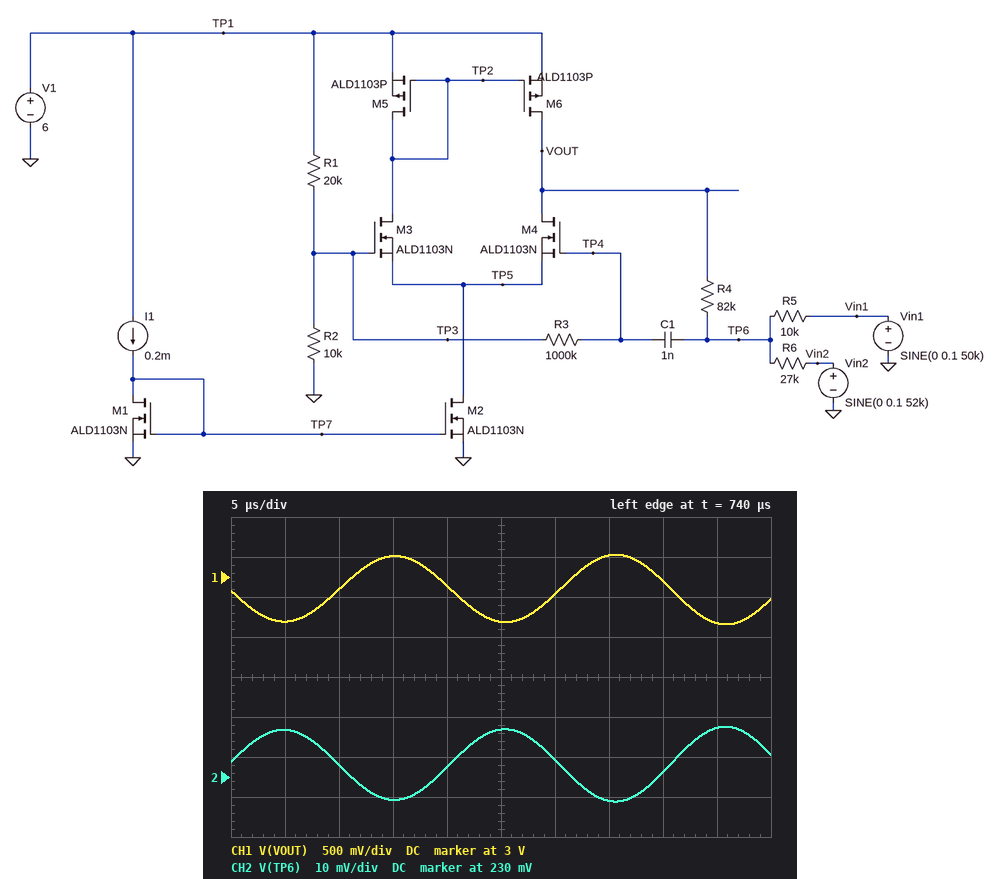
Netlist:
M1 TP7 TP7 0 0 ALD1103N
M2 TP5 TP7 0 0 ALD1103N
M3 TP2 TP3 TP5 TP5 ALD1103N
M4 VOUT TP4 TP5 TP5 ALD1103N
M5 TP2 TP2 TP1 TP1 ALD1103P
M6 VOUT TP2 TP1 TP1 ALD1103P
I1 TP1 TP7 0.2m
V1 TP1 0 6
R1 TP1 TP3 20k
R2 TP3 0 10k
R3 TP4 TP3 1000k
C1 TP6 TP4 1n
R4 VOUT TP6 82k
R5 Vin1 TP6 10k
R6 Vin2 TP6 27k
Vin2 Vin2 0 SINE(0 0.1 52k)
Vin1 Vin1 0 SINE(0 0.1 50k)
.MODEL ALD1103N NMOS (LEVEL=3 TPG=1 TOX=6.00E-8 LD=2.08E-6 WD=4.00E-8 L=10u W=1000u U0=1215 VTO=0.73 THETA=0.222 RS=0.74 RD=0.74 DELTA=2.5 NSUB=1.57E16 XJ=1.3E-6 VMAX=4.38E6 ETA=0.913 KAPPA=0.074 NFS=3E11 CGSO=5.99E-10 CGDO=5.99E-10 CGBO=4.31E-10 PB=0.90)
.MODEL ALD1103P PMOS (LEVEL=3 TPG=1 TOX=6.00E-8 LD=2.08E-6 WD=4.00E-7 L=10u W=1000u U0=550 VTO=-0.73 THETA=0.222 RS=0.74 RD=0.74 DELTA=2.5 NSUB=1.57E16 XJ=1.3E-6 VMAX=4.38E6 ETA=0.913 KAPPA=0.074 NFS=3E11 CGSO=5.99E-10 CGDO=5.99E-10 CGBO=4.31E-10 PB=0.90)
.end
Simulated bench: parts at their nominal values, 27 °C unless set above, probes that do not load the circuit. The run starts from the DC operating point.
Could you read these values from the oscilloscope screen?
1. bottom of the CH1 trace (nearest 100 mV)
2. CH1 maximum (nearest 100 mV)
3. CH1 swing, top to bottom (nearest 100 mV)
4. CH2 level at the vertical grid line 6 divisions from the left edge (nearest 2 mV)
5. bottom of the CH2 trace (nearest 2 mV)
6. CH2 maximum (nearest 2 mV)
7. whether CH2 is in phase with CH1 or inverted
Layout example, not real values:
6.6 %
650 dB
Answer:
2.4 V
3.3 V
900 mV
234 mV
224 mV
242 mV
inverted
